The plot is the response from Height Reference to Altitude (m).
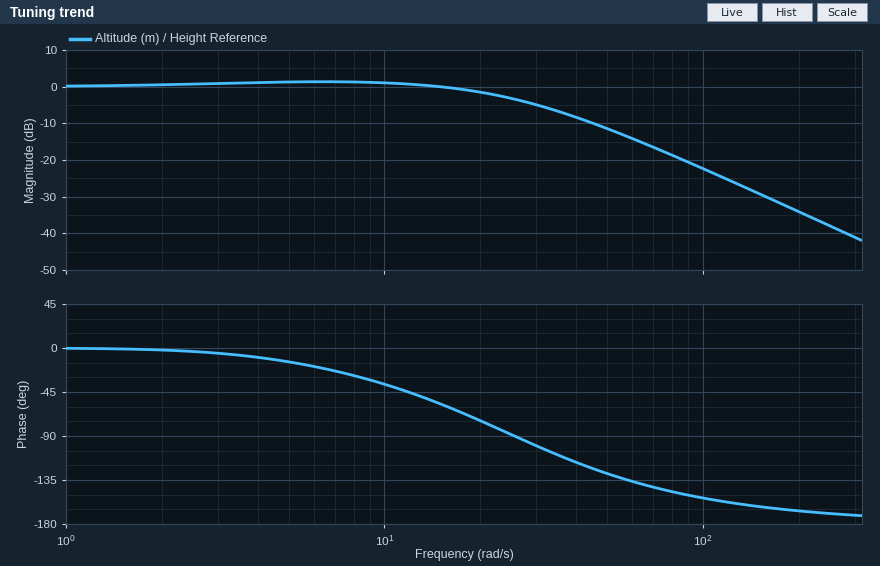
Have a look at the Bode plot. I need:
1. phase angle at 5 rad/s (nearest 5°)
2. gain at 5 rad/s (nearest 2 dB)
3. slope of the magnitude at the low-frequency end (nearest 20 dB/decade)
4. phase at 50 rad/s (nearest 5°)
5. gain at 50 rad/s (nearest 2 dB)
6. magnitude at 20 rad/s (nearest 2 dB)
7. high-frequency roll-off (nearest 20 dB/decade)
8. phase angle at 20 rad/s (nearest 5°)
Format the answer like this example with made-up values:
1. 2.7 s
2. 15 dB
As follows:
1. -15°
2. 2 dB
3. 0 dB/decade
4. -130°
5. -12 dB
6. -2 dB
7. -40 dB/decade
8. -75°
